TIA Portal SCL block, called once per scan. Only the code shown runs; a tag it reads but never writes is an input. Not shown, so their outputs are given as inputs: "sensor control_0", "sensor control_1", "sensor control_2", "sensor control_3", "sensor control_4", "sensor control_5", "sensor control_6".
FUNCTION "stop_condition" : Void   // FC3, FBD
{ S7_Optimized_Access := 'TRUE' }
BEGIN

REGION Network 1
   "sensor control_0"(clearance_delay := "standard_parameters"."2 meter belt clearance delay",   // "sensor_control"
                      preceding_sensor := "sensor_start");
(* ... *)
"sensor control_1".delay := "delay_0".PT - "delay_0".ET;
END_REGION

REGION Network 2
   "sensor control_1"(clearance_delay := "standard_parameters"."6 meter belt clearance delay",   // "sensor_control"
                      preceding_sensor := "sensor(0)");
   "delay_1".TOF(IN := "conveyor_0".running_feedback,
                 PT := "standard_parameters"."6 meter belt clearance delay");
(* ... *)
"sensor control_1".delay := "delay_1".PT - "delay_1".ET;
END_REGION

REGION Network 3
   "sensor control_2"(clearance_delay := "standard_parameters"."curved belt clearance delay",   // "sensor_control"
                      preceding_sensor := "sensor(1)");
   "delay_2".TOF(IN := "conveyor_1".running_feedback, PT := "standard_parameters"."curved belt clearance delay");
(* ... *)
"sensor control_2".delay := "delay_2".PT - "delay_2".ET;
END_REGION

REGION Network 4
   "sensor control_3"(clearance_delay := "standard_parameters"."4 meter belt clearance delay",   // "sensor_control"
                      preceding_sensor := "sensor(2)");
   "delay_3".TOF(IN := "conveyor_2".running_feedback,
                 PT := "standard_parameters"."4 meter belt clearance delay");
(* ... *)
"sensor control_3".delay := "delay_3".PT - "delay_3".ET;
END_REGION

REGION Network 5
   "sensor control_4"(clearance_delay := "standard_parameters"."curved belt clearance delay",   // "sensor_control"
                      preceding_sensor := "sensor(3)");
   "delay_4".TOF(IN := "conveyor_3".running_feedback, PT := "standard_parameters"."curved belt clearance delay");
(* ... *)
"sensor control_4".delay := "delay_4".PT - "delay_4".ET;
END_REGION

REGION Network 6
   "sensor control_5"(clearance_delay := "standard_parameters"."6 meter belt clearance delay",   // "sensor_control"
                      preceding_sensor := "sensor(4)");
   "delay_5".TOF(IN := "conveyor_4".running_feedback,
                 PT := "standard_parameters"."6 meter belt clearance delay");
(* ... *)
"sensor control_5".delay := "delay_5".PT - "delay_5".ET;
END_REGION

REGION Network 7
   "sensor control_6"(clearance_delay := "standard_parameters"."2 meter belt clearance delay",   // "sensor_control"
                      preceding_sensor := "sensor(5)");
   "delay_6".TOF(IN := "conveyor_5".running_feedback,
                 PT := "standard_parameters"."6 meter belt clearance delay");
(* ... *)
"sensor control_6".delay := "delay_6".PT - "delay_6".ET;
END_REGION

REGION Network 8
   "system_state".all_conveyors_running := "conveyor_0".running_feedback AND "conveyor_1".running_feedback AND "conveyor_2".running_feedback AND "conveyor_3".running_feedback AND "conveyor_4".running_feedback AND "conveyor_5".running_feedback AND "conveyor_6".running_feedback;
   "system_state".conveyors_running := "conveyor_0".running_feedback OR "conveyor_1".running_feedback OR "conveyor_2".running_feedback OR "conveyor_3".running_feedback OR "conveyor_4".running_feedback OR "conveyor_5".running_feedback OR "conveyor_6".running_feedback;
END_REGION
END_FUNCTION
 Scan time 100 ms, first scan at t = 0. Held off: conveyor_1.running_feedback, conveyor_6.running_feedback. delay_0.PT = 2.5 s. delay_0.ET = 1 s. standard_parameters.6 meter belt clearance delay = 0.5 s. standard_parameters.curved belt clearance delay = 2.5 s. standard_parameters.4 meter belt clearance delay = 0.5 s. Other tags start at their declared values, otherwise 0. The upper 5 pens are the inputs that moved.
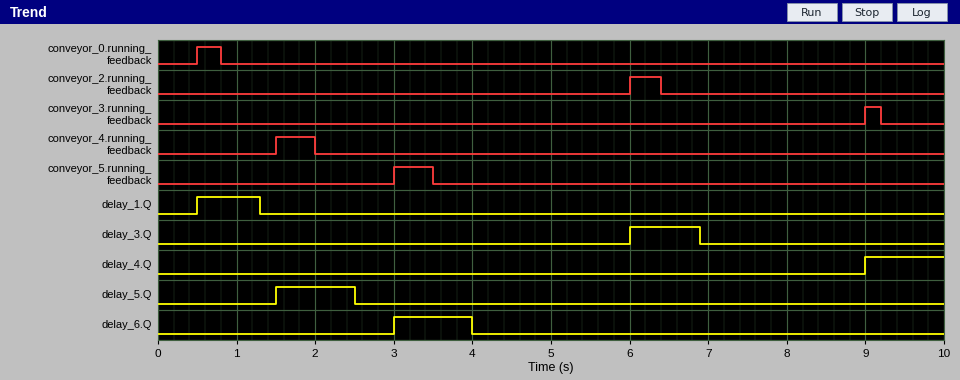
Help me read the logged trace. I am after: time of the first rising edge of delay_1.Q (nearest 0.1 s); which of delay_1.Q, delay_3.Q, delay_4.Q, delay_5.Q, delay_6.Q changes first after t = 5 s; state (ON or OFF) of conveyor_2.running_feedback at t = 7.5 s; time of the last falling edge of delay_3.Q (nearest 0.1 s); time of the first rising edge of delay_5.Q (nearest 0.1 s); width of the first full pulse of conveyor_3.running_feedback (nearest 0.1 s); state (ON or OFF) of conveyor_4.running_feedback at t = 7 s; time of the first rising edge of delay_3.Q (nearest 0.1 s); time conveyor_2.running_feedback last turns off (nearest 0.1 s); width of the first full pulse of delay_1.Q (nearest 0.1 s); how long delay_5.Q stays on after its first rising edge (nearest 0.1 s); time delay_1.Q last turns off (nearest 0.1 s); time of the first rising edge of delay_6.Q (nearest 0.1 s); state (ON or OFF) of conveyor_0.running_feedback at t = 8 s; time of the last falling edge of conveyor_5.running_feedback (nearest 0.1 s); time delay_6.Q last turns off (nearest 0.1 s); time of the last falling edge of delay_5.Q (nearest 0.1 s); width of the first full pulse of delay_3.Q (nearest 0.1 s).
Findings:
0.5 s
delay_3.Q
OFF
6.9 s
1.5 s
0.2 s
OFF
6.0 s
6.4 s
0.8 s
1.0 s
1.3 s
3.0 s
OFF
3.5 s
4.0 s
2.5 s
0.9 s
